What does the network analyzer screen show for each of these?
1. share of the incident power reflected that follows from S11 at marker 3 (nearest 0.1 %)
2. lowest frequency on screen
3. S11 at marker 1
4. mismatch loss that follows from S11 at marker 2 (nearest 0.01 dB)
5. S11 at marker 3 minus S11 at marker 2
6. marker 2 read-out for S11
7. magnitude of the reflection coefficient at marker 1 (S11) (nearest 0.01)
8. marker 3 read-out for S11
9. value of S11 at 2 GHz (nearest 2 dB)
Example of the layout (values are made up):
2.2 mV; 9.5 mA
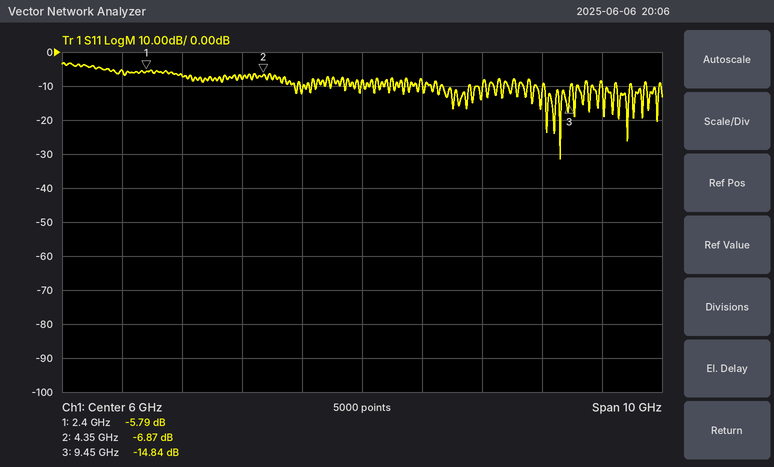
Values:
3.3 %; 1 GHz; -5.79 dB; 1.00 dB; -7.97 dB; -6.87 dB; 0.51; -14.84 dB; -6 dB
